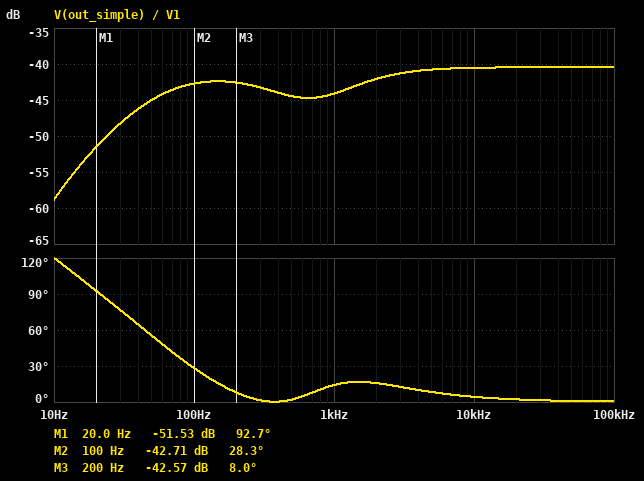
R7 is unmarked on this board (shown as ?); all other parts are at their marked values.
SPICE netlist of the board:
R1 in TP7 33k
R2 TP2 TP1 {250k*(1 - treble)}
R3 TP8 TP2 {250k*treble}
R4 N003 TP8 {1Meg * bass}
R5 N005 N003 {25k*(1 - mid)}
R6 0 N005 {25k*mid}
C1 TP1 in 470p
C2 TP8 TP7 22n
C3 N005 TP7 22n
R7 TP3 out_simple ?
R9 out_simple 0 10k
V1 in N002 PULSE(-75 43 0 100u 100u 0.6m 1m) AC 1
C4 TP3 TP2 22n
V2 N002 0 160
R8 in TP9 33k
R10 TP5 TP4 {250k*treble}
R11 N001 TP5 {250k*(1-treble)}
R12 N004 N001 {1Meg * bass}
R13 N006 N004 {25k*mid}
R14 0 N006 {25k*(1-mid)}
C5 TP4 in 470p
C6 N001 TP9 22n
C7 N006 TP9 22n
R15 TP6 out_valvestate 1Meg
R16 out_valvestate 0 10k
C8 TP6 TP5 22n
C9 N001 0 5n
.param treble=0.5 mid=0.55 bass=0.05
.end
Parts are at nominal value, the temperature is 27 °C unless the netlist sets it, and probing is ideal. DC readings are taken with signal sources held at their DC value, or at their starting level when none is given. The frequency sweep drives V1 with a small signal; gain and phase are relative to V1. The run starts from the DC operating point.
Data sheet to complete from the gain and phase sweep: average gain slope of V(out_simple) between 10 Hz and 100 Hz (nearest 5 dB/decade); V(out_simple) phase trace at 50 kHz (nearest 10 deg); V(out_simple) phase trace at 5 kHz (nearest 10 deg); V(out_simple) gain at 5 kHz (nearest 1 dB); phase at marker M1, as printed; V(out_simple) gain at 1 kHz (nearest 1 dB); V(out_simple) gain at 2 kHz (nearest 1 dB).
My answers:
15 dB/decade
0 deg
10 deg
-41 dB
92.7 deg
-44 dB
-42 dB
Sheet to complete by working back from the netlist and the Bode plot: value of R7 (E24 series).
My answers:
620 kΩ
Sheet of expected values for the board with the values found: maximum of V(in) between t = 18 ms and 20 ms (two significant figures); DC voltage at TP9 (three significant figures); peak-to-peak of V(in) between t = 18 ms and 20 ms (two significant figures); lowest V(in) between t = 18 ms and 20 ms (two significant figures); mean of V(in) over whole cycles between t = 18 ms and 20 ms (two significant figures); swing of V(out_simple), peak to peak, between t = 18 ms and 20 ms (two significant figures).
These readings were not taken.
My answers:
200 V
85.0 V
120 V
85 V
170 V
1.2 V
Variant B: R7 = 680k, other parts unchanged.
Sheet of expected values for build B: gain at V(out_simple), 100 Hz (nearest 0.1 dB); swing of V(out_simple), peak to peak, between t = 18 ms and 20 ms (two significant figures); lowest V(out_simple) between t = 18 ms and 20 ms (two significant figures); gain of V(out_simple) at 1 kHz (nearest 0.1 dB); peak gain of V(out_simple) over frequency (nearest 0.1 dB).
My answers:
-43.3 dB
1.1 V
-700 mV
-44.8 dB
-41.2 dB
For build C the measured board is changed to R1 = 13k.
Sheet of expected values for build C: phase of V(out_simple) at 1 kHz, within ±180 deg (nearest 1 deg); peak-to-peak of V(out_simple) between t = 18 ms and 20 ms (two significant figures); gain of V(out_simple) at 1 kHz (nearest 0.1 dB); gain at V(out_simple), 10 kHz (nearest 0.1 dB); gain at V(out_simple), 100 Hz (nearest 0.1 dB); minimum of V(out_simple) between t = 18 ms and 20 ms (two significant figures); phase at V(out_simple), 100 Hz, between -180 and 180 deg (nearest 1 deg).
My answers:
5 deg
1.3 V
-41.2 dB
-39.2 dB
-40.6 dB
-900 mV
39 deg
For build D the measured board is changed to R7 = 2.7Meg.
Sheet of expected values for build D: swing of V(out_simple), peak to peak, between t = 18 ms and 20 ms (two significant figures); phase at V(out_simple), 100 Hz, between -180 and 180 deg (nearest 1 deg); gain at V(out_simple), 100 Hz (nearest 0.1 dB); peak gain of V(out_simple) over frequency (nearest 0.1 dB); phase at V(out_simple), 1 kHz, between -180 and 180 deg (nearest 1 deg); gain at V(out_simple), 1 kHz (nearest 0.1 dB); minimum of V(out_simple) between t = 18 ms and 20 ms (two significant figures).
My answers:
290 mV
23 deg
-53.8 dB
-52.5 dB
11 deg
-55.7 dB
-190 mV
